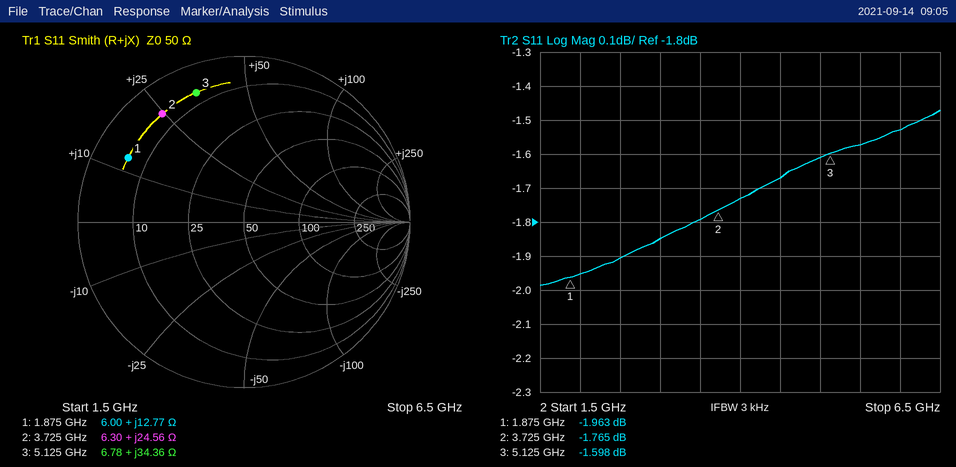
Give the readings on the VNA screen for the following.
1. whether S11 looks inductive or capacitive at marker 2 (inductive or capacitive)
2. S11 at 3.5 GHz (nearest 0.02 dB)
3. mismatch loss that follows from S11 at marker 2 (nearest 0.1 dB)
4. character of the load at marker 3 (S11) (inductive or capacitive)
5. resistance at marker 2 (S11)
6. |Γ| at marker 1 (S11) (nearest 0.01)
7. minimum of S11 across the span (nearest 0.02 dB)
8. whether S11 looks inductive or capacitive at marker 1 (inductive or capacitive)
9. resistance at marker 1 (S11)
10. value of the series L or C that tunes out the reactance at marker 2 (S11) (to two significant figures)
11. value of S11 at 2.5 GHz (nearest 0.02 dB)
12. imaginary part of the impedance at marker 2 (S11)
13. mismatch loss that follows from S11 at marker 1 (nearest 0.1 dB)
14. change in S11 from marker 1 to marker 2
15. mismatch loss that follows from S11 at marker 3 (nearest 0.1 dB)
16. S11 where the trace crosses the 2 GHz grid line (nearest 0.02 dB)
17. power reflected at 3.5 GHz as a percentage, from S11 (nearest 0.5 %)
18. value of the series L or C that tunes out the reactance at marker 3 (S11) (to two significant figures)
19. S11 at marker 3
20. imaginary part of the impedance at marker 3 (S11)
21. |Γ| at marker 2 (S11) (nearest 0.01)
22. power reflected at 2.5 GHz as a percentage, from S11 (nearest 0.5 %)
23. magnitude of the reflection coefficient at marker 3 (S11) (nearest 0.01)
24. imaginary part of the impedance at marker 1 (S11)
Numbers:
inductive
-1.80 dB
4.8 dB
inductive
6.30 Ω
0.80
-1.98 dB
inductive
6.00 Ω
1.7 pF
-1.90 dB
+24.56 Ω
4.4 dB
0.198 dB
5.1 dB
-1.96 dB
66.0 %
900 fF
-1.598 dB
+34.36 Ω
0.82
64.5 %
0.83
+12.77 Ω
